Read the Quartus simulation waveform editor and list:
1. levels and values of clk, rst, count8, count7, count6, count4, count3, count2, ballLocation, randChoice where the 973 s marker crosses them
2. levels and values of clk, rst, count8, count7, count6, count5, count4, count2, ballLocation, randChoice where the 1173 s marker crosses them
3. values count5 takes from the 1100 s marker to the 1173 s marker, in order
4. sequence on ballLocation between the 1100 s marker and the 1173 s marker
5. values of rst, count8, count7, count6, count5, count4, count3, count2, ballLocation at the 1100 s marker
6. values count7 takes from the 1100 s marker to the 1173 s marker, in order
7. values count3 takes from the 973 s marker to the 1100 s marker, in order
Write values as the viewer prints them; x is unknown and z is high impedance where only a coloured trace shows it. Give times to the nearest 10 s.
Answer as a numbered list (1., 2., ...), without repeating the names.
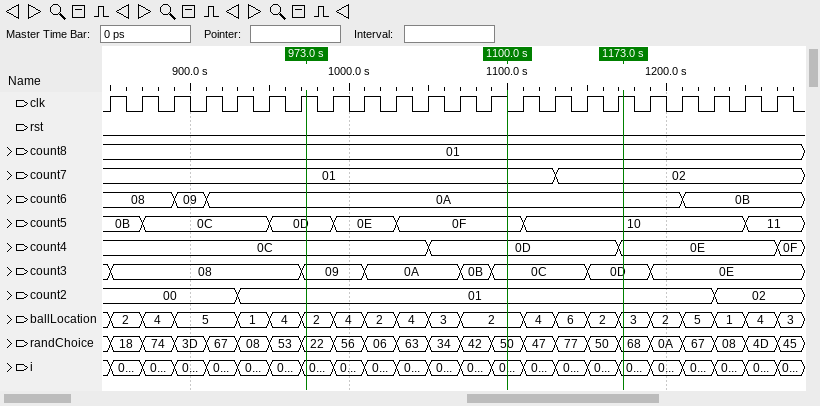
1. clk=1, rst=0, count8=01, count7=01, count6=0A, count4=0C, count3=09, count2=01, ballLocation=2, randChoice=22
2. clk=1, rst=0, count8=01, count7=02, count6=0A, count5=10, count4=0E, count2=01, ballLocation=3, randChoice=68
3. 0F, 10
4. 2, 4, 6, 2, 3
5. rst=0, count8=01, count7=01, count6=0A, count5=0F, count4=0D, count3=0C, count2=01, ballLocation=2
6. 01, 02
7. 09, 0A, 0B, 0C
